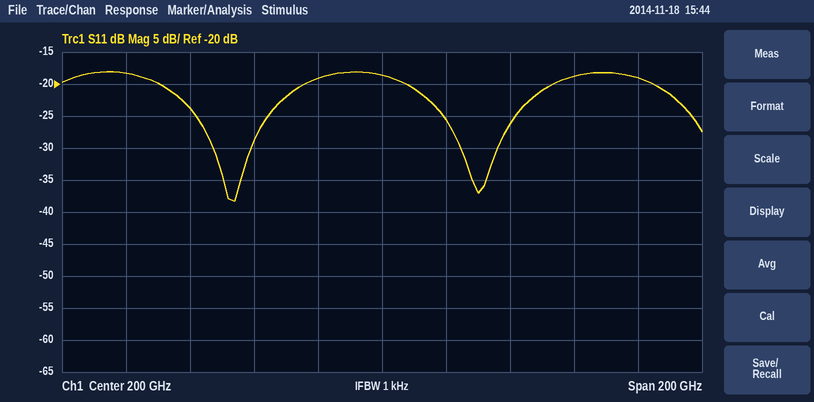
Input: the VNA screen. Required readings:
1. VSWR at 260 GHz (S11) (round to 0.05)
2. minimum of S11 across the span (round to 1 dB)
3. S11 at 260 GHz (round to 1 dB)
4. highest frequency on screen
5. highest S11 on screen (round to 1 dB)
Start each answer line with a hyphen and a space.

- 1.25
- -38 dB
- -19 dB
- 300 GHz
- -18 dB
